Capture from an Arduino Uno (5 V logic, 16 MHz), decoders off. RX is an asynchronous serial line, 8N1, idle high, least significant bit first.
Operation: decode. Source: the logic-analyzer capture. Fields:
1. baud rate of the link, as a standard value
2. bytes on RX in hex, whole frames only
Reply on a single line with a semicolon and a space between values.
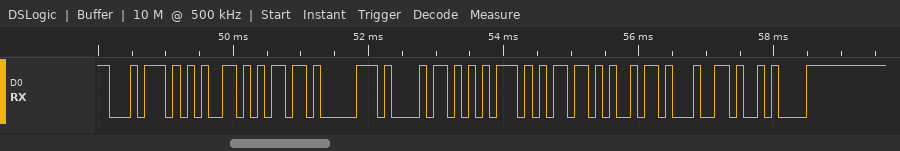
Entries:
9600 baud; 0x74 0x65 0x6D 0x70 0x68 0x75 0x6D 0x69 0x64 0x0A
